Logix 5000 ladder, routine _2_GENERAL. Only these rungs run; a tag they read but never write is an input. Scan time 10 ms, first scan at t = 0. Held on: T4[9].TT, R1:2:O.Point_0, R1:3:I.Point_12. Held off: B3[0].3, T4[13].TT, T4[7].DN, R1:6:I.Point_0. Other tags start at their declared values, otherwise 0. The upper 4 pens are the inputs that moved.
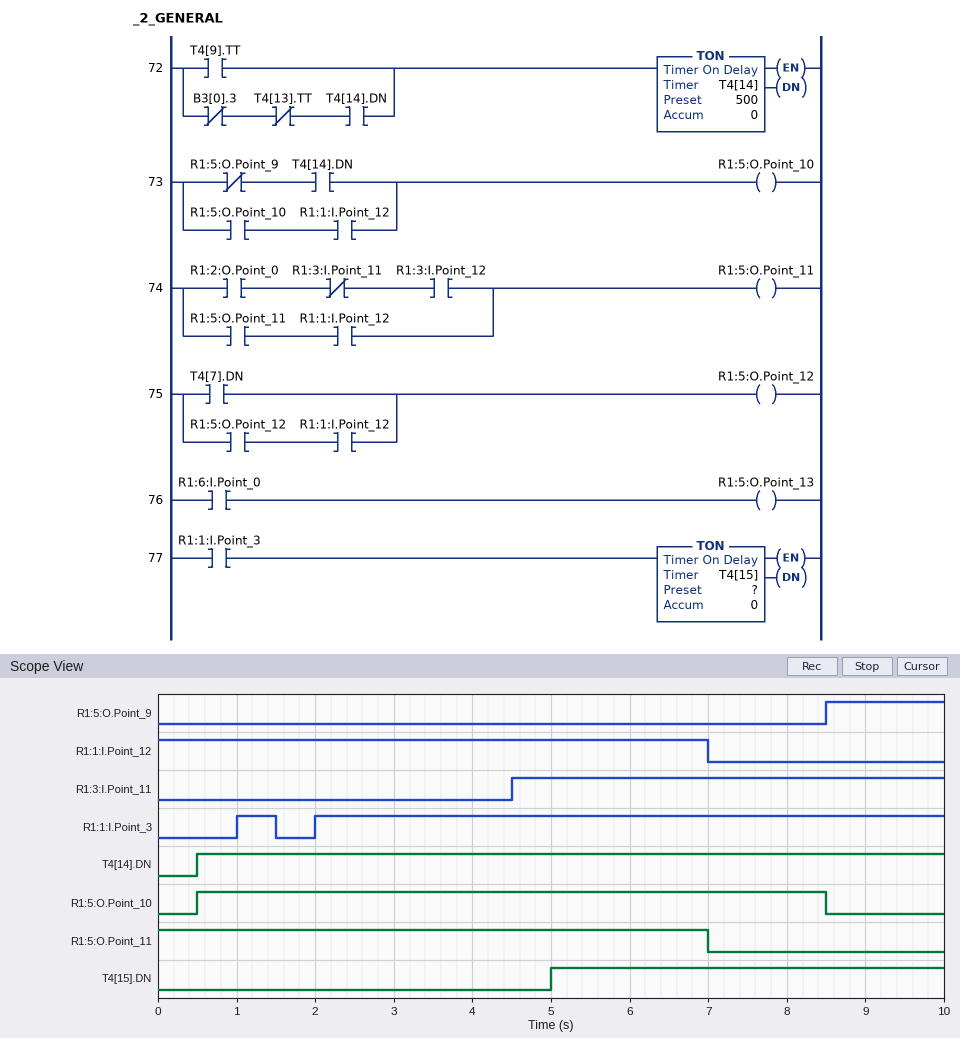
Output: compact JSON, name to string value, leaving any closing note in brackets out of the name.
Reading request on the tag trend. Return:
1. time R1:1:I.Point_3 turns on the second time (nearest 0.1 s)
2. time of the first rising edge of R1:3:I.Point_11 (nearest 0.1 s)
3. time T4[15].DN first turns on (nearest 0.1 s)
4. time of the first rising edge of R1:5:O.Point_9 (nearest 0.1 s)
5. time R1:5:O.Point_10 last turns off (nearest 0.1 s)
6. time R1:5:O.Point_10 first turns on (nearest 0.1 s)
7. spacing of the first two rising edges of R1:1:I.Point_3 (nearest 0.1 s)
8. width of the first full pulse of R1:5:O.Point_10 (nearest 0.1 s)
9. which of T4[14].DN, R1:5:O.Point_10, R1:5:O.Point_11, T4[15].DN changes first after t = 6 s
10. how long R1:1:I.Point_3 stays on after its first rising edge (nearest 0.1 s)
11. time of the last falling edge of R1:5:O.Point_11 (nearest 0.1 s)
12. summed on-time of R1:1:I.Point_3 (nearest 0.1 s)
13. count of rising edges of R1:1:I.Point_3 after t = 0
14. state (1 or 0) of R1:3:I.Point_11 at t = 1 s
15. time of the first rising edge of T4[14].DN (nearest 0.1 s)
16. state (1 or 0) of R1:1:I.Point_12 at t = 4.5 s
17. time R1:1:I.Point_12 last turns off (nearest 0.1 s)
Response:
{"time R1:1:I.Point_3 turns on the second time": "2.0 s", "time of the first rising edge of R1:3:I.Point_11": "4.5 s", "time T4[15].DN first turns on": "5.0 s", "time of the first rising edge of R1:5:O.Point_9": "8.5 s", "time R1:5:O.Point_10 last turns off": "8.5 s", "time R1:5:O.Point_10 first turns on": "0.5 s", "spacing of the first two rising edges of R1:1:I.Point_3": "1.0 s", "width of the first full pulse of R1:5:O.Point_10": "8.0 s", "which of T4[14].DN, R1:5:O.Point_10, R1:5:O.Point_11, T4[15].DN changes first after t = 6 s": "R1:5:O.Point_11", "how long R1:1:I.Point_3 stays on after its first rising edge": "0.5 s", "time of the last falling edge of R1:5:O.Point_11": "7.0 s", "summed on-time of R1:1:I.Point_3": "8.5 s", "count of rising edges of R1:1:I.Point_3 after t = 0": "2", "state (1 or 0) of R1:3:I.Point_11 at t = 1 s": "0", "time of the first rising edge of T4[14].DN": "0.5 s", "state (1 or 0) of R1:1:I.Point_12 at t = 4.5 s": "1", "time R1:1:I.Point_12 last turns off": "7.0 s"}
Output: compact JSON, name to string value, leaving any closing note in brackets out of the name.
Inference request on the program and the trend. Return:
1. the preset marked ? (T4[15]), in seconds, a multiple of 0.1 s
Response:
{"the preset marked ? (T4[15]), in seconds, a multiple of 0.1 s": "3.0 s"}
